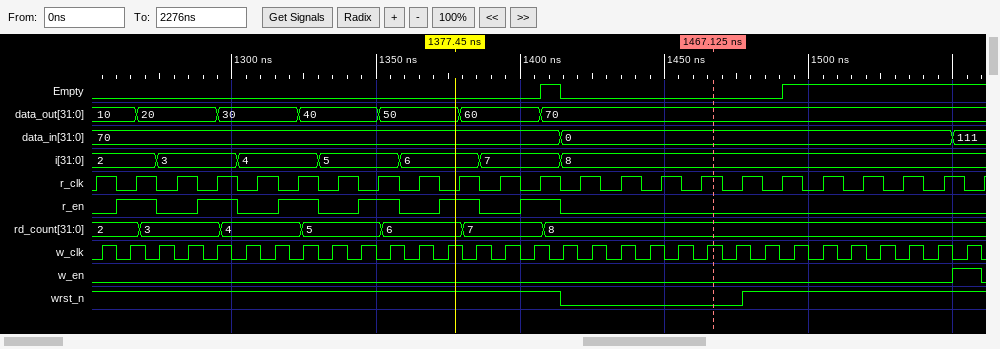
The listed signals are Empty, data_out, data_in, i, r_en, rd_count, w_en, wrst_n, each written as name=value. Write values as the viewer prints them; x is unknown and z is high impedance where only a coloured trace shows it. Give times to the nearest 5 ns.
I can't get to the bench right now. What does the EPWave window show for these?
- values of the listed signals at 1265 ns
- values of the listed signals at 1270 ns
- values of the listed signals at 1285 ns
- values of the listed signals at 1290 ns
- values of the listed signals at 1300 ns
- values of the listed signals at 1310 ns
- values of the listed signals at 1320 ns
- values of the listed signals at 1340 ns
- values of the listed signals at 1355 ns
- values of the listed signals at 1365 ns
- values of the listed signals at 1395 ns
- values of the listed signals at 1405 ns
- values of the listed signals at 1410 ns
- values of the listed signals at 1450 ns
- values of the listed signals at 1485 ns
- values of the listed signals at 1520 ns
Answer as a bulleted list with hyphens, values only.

- Empty=0, data_out=10, data_in=70, i=2, r_en=1, rd_count=2, w_en=0, wrst_n=1
- Empty=0, data_out=20, data_in=70, i=2, r_en=1, rd_count=3, w_en=0, wrst_n=1
- Empty=0, data_out=20, data_in=70, i=3, r_en=0, rd_count=3, w_en=0, wrst_n=1
- Empty=0, data_out=20, data_in=70, i=3, r_en=1, rd_count=3, w_en=0, wrst_n=1
- Empty=0, data_out=30, data_in=70, i=3, r_en=1, rd_count=4, w_en=0, wrst_n=1
- Empty=0, data_out=30, data_in=70, i=4, r_en=0, rd_count=4, w_en=0, wrst_n=1
- Empty=0, data_out=30, data_in=70, i=4, r_en=1, rd_count=4, w_en=0, wrst_n=1
- Empty=0, data_out=40, data_in=70, i=5, r_en=0, rd_count=5, w_en=0, wrst_n=1
- Empty=0, data_out=50, data_in=70, i=5, r_en=1, rd_count=6, w_en=0, wrst_n=1
- Empty=0, data_out=50, data_in=70, i=6, r_en=0, rd_count=6, w_en=0, wrst_n=1
- Empty=0, data_out=60, data_in=70, i=7, r_en=0, rd_count=7, w_en=0, wrst_n=1
- Empty=0, data_out=60, data_in=70, i=7, r_en=1, rd_count=7, w_en=0, wrst_n=1
- Empty=1, data_out=70, data_in=70, i=7, r_en=1, rd_count=8, w_en=0, wrst_n=1
- Empty=0, data_out=70, data_in=0, i=8, r_en=0, rd_count=8, w_en=0, wrst_n=0
- Empty=0, data_out=70, data_in=0, i=8, r_en=0, rd_count=8, w_en=0, wrst_n=1
- Empty=1, data_out=70, data_in=0, i=8, r_en=0, rd_count=8, w_en=0, wrst_n=1
